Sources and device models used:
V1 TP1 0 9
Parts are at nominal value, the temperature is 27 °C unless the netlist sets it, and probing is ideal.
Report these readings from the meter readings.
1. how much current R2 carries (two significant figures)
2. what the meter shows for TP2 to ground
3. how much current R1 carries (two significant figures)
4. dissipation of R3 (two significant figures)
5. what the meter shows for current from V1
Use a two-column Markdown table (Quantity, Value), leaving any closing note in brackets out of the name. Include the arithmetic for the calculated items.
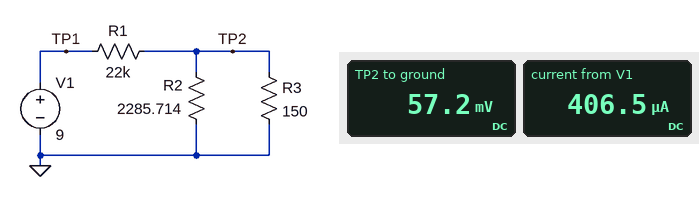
| Quantity | Value |
|---|---|
| how much current R2 carries | (57.2 mV) / 2.286 kΩ = 25 µA |
| what the meter shows for TP2 to ground | 57.2 mV |
| how much current R1 carries | (9 V - 57.2 mV) / 22 kΩ = 410 µA |
| dissipation of R3 | (57.2 mV)^2 / 150 Ω = 22 µW |
| what the meter shows for current from V1 | 406.5 µA |
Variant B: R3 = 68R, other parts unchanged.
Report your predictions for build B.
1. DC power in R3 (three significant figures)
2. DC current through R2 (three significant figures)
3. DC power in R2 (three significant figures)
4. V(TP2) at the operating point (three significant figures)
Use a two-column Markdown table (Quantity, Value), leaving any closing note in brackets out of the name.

| Quantity | Value |
|---|---|
| DC power in R3 | 10.7 µW |
| DC current through R2 | 11.8 µA |
| DC power in R2 | 317 nW |
| V(TP2) at the operating point | 26.9 mV |
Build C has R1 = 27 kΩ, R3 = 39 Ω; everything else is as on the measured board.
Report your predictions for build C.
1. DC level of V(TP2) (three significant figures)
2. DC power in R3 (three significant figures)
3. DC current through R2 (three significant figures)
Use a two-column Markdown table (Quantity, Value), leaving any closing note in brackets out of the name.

| Quantity | Value |
|---|---|
| DC level of V(TP2) | 12.8 mV |
| DC power in R3 | 4.18 µW |
| DC current through R2 | 5.58 µA |
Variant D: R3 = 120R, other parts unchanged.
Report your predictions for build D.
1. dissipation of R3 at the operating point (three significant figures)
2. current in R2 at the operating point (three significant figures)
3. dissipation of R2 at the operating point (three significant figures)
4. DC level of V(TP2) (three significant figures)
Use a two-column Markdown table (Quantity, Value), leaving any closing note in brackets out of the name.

| Quantity | Value |
|---|---|
| dissipation of R3 at the operating point | 17.9 µW |
| current in R2 at the operating point | 20.3 µA |
| dissipation of R2 at the operating point | 942 nW |
| DC level of V(TP2) | 46.4 mV |
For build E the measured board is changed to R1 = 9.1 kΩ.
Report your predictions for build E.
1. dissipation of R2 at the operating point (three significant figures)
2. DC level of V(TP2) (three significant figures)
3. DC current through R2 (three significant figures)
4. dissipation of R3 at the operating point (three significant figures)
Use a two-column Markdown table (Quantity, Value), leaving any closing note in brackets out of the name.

| Quantity | Value |
|---|---|
| dissipation of R2 at the operating point | 8.22 µW |
| DC level of V(TP2) | 137 mV |
| DC current through R2 | 60.0 µA |
| dissipation of R3 at the operating point | 125 µW |
